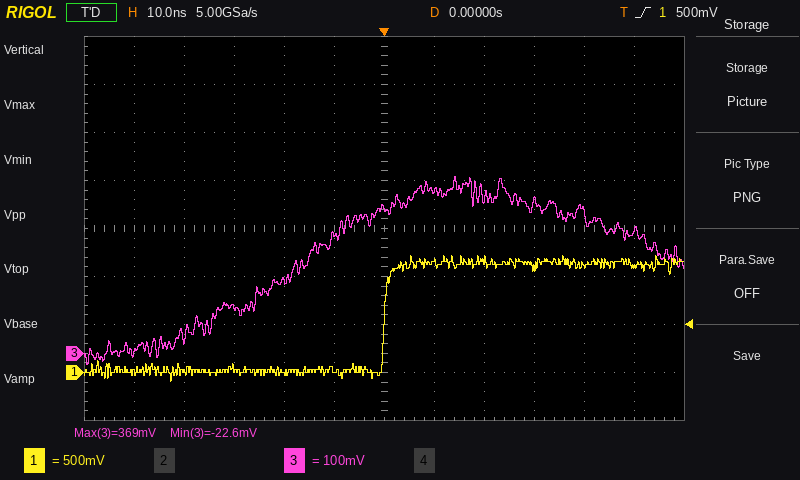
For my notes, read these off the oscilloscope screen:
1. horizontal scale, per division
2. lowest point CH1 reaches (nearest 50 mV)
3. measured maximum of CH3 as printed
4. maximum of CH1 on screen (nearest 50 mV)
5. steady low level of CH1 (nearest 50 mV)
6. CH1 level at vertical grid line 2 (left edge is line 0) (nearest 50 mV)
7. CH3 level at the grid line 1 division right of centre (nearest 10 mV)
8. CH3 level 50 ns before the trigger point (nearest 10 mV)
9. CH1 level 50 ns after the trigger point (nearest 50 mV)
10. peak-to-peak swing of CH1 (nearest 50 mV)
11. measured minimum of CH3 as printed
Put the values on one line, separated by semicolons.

10 ns; -100 mV; 369 mV; 1.20 V; 0 mV; 0 mV; 340 mV; 0 mV; 1.10 V; 1.30 V; -22.6 mV
